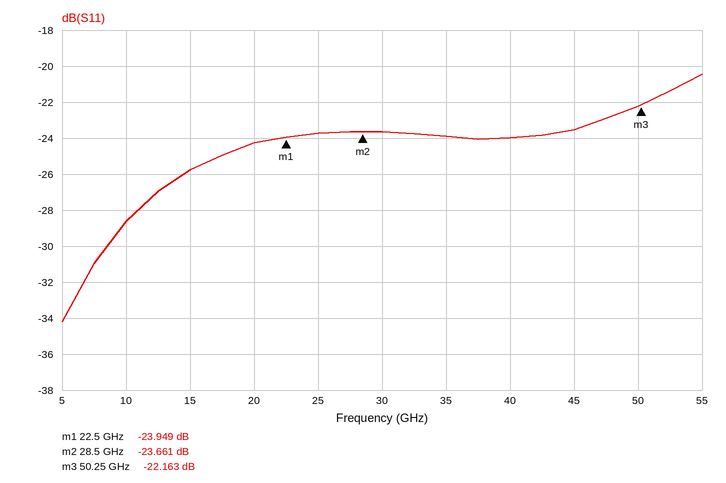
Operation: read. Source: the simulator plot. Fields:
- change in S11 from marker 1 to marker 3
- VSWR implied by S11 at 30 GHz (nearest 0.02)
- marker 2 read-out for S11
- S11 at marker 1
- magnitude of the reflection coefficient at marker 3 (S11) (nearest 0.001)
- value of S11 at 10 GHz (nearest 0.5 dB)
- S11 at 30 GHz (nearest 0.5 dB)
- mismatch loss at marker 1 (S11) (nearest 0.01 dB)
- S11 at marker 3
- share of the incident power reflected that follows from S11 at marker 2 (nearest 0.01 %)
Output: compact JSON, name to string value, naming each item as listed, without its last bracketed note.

{"change in S11 from marker 1 to marker 3": "1.786 dB", "VSWR implied by S11 at 30 GHz": "1.14", "marker 2 read-out for S11": "-23.661 dB", "S11 at marker 1": "-23.949 dB", "magnitude of the reflection coefficient at marker 3 (S11)": "0.078", "value of S11 at 10 GHz": "-28.5 dB", "S11 at 30 GHz": "-23.5 dB", "mismatch loss at marker 1 (S11)": "0.02 dB", "S11 at marker 3": "-22.163 dB", "share of the incident power reflected that follows from S11 at marker 2": "0.43 %"}
